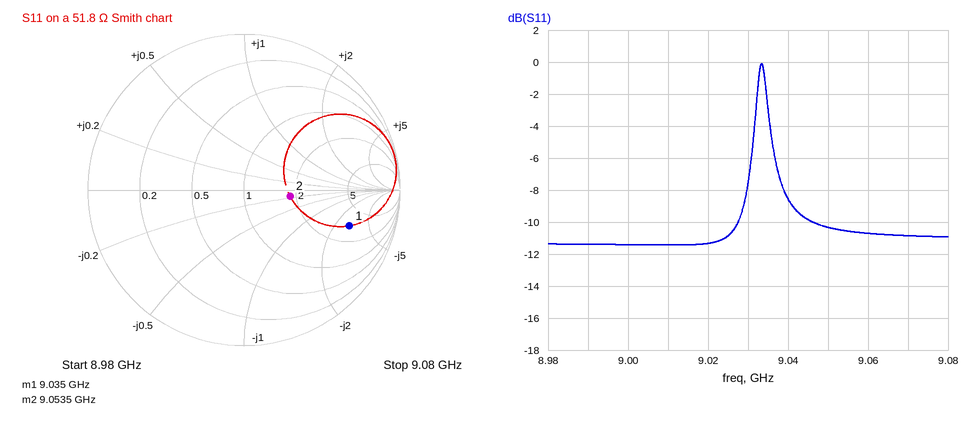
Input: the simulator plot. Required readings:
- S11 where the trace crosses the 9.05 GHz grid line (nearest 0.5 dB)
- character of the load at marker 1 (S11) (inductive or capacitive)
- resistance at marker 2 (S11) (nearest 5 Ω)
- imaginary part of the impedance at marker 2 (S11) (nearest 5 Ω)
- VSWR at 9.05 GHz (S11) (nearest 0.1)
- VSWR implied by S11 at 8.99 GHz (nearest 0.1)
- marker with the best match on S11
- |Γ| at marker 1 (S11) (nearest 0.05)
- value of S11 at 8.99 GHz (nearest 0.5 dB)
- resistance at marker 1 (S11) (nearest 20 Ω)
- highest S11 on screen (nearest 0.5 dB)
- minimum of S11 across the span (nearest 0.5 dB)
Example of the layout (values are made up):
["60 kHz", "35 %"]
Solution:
["-10.5 dB", "capacitive", "95 Ω", "-10 Ω", "1.9", "1.7", "marker 2", "0.70", "-11.5 dB", "160 Ω", "0.0 dB", "-11.5 dB"]
